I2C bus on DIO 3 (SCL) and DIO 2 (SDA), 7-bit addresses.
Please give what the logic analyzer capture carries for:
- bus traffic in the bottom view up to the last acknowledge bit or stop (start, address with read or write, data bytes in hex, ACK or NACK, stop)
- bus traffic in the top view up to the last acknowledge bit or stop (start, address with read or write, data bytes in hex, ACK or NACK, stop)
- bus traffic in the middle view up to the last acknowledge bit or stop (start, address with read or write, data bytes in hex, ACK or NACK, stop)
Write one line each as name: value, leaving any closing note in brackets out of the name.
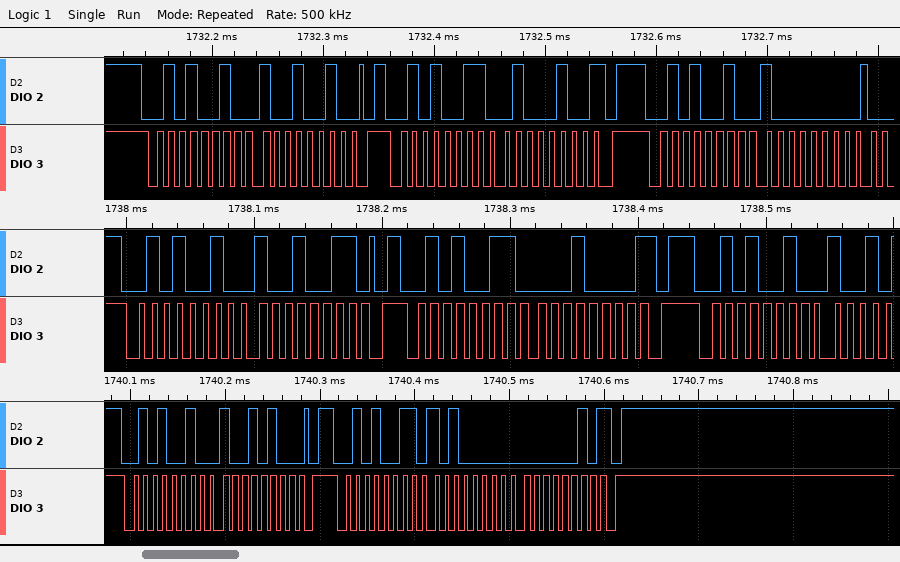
bus traffic in the bottom view up to the last acknowledge bit or stop: start, address 29 write ACK, 94 ACK, stop, start, address 29 read ACK, A0 ACK, 02 NACK, stop
bus traffic in the top view up to the last acknowledge bit or stop: start, address 29 write ACK, 92 ACK, stop, start, address 29 read ACK, 44 NACK, stop, start, address 29 write ACK, 80 ACK
bus traffic in the middle view up to the last acknowledge bit or stop: start, address 29 write ACK, 93 ACK, stop, start, address 29 read ACK, 10 NACK, stop, start, address 29 write ACK
